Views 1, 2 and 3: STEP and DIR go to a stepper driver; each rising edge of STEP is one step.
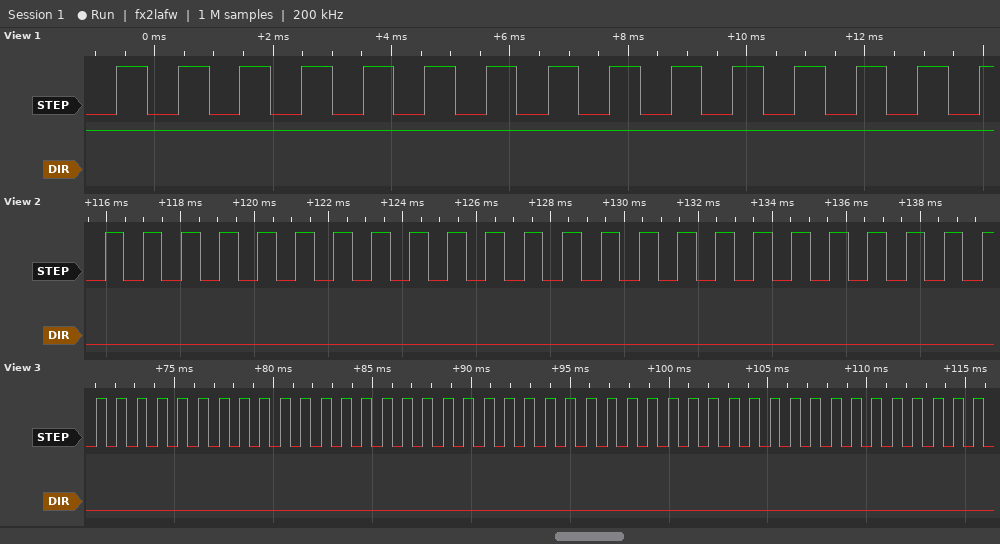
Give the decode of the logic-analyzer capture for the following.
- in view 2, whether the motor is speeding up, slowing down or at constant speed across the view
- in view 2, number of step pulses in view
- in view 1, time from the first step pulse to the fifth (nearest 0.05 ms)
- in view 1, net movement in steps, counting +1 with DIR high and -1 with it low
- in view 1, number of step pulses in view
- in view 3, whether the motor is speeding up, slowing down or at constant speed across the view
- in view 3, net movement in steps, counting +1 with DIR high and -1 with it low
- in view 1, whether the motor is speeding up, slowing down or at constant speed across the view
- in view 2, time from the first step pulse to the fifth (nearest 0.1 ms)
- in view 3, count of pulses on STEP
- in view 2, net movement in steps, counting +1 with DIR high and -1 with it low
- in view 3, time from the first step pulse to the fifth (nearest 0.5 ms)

constant speed
24
4.15 ms
+15
15
constant speed
-44
constant speed
4.1 ms
44
-24
4.0 ms
